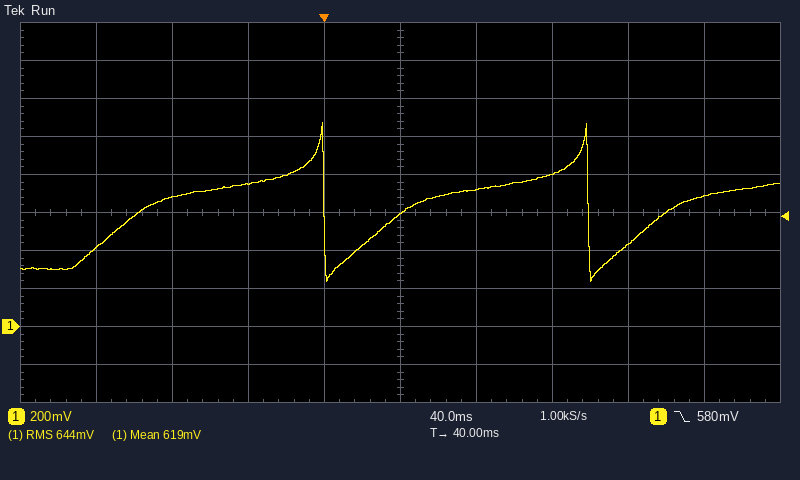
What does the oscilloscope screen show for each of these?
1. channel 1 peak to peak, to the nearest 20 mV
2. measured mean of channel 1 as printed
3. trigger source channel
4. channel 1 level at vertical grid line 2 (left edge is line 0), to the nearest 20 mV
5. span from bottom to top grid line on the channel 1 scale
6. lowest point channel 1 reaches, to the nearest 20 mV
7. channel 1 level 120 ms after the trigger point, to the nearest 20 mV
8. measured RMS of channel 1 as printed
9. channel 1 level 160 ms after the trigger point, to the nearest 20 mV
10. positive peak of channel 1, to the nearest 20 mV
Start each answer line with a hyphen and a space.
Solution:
- 840 mV
- 619 mV
- channel 1
- 680 mV
- 2 V
- 240 mV
- 800 mV
- 644 mV
- 440 mV
- 1.08 V
